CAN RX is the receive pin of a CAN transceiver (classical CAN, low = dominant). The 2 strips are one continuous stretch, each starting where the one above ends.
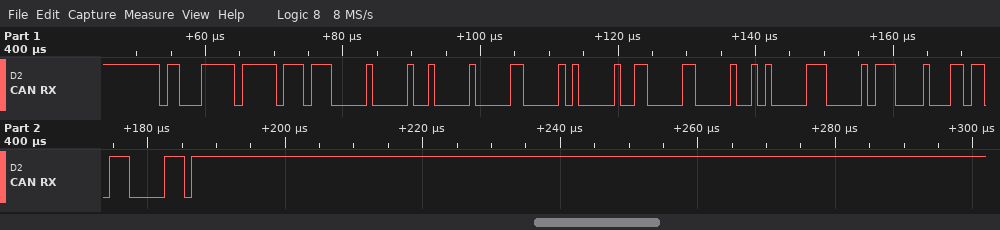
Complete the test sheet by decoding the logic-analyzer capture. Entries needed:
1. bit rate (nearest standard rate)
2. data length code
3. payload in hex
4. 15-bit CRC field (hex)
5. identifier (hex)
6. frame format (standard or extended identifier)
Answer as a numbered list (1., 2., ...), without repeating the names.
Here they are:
1. 1000 kbit/s
2. 8
3. 01 02 03 04 05 06 07 08
4. 0x6DC1
5. 0x18FFEE00
6. extended
